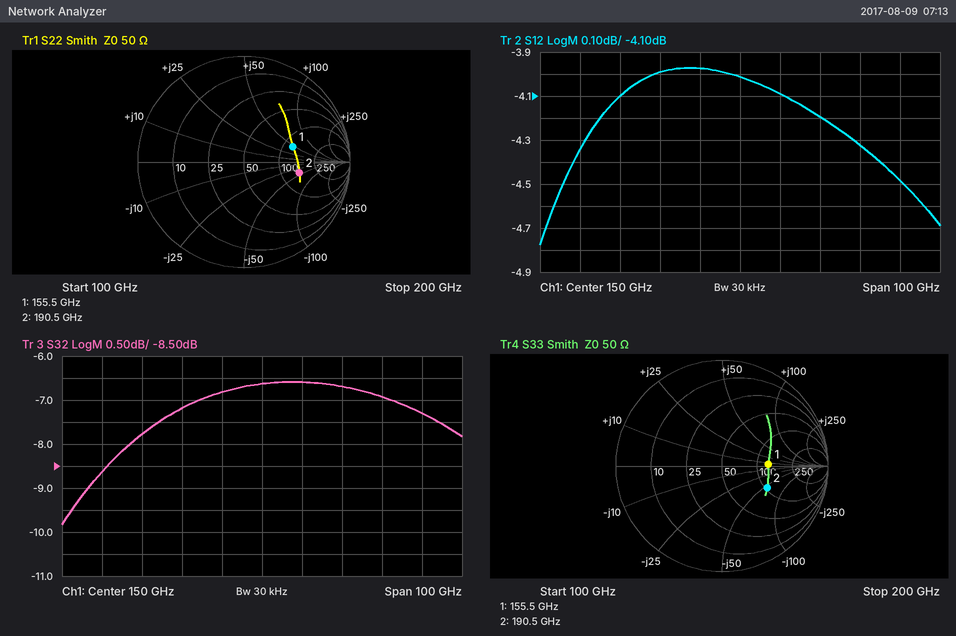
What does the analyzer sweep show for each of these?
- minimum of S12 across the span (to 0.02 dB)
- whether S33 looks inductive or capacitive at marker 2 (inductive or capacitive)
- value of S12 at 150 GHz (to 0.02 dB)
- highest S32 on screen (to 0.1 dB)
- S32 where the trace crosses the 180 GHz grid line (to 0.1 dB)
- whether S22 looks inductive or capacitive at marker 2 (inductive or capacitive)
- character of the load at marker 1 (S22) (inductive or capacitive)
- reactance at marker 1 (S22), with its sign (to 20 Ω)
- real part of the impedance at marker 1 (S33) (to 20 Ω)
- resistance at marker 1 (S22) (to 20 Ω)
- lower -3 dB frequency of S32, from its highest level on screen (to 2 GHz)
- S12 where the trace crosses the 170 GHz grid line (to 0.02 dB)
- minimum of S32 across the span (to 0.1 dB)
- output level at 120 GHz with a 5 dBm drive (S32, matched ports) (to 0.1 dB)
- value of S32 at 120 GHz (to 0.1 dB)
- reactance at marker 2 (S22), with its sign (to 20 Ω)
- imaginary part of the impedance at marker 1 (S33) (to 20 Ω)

-4.78 dB
capacitive
-4.02 dB
-6.6 dB
-6.9 dB
capacitive
inductive
+40 Ω
120 Ω
120 Ω
102 GHz
-4.20 dB
-9.8 dB
-2.8 dBm
-7.8 dB
-40 Ω
0 Ω
